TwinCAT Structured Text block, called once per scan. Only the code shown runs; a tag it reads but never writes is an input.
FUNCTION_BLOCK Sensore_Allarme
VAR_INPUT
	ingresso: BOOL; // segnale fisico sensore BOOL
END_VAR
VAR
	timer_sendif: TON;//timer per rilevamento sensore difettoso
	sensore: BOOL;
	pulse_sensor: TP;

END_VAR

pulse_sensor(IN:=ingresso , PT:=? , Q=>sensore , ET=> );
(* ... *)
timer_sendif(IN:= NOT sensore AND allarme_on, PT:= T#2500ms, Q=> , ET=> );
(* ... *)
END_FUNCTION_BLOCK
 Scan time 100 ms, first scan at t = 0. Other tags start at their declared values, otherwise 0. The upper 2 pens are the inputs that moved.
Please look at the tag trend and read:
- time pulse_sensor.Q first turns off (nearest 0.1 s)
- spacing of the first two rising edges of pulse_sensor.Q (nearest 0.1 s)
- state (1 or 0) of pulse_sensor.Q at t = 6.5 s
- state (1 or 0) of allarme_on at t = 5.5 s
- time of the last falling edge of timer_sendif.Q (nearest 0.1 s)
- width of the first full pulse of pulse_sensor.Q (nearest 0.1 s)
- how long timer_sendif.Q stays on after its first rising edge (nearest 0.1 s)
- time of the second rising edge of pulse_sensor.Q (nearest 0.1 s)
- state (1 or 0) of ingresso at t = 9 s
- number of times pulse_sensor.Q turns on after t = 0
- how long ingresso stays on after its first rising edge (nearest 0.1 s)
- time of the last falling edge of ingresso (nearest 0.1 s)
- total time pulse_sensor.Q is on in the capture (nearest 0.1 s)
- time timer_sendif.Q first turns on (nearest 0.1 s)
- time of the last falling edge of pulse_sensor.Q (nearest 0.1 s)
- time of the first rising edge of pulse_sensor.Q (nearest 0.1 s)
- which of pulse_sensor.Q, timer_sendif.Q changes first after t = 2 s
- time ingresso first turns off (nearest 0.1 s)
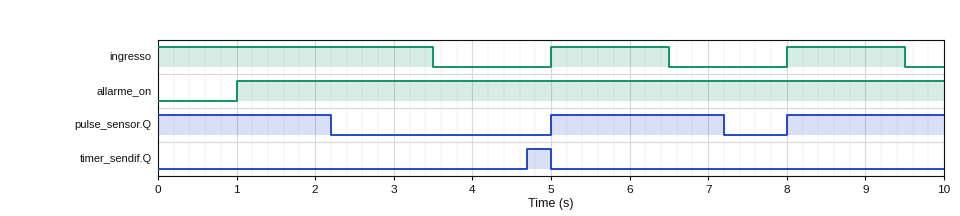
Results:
2.2 s
3.0 s
1
1
5.0 s
2.2 s
0.3 s
8.0 s
1
2
1.5 s
9.5 s
6.4 s
4.7 s
7.2 s
5.0 s
pulse_sensor.Q
3.5 s
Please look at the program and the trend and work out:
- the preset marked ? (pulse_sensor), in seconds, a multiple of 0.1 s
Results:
2.2 s
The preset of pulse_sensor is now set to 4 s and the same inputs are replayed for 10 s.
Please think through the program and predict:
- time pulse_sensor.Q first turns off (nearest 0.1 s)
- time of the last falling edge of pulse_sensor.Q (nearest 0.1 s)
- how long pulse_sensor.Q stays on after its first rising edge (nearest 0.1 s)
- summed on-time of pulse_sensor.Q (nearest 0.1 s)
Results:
4.0 s
9.0 s
4.0 s
8.0 s
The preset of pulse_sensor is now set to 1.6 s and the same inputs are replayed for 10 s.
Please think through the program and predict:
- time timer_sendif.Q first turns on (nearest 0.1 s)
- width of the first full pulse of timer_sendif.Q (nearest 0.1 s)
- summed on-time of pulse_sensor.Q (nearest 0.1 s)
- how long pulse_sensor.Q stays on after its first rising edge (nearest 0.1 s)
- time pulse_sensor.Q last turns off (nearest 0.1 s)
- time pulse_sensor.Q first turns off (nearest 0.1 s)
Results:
4.1 s
0.9 s
4.8 s
1.6 s
9.6 s
1.6 s
